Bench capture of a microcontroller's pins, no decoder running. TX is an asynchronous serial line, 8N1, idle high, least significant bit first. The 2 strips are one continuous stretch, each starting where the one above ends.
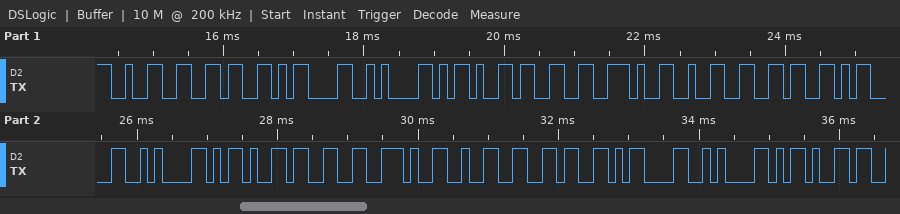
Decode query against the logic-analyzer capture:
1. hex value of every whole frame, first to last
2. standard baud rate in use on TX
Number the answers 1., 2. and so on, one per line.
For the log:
1. 32 36 0D 0A 2D 33 2E 32 36 0D 0A 2D 33 2E 32 36 0D 0A 2D
2. 9600 baud
